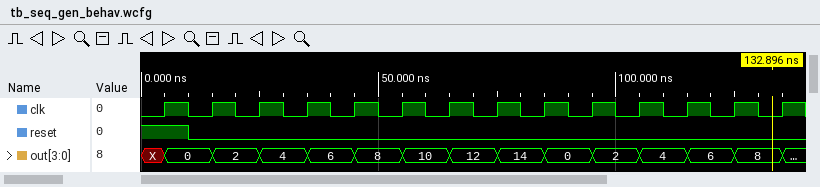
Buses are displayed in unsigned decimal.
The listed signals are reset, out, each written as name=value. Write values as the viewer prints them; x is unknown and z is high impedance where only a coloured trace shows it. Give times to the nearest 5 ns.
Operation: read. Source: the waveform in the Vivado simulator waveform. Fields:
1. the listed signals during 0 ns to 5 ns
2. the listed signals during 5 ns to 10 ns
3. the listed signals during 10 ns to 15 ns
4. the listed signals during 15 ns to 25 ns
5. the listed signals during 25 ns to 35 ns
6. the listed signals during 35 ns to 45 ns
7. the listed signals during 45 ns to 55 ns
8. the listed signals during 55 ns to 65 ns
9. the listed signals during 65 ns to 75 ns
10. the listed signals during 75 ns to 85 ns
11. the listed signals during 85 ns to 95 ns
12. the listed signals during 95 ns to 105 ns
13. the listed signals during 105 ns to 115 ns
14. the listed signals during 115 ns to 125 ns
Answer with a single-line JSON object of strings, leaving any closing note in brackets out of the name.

{"the listed signals during 0 ns to 5 ns": "reset=1, out=X", "the listed signals during 5 ns to 10 ns": "reset=1, out=0", "the listed signals during 10 ns to 15 ns": "reset=0, out=0", "the listed signals during 15 ns to 25 ns": "reset=0, out=2", "the listed signals during 25 ns to 35 ns": "reset=0, out=4", "the listed signals during 35 ns to 45 ns": "reset=0, out=6", "the listed signals during 45 ns to 55 ns": "reset=0, out=8", "the listed signals during 55 ns to 65 ns": "reset=0, out=10", "the listed signals during 65 ns to 75 ns": "reset=0, out=12", "the listed signals during 75 ns to 85 ns": "reset=0, out=14", "the listed signals during 85 ns to 95 ns": "reset=0, out=0", "the listed signals during 95 ns to 105 ns": "reset=0, out=2", "the listed signals during 105 ns to 115 ns": "reset=0, out=4", "the listed signals during 115 ns to 125 ns": "reset=0, out=6"}
